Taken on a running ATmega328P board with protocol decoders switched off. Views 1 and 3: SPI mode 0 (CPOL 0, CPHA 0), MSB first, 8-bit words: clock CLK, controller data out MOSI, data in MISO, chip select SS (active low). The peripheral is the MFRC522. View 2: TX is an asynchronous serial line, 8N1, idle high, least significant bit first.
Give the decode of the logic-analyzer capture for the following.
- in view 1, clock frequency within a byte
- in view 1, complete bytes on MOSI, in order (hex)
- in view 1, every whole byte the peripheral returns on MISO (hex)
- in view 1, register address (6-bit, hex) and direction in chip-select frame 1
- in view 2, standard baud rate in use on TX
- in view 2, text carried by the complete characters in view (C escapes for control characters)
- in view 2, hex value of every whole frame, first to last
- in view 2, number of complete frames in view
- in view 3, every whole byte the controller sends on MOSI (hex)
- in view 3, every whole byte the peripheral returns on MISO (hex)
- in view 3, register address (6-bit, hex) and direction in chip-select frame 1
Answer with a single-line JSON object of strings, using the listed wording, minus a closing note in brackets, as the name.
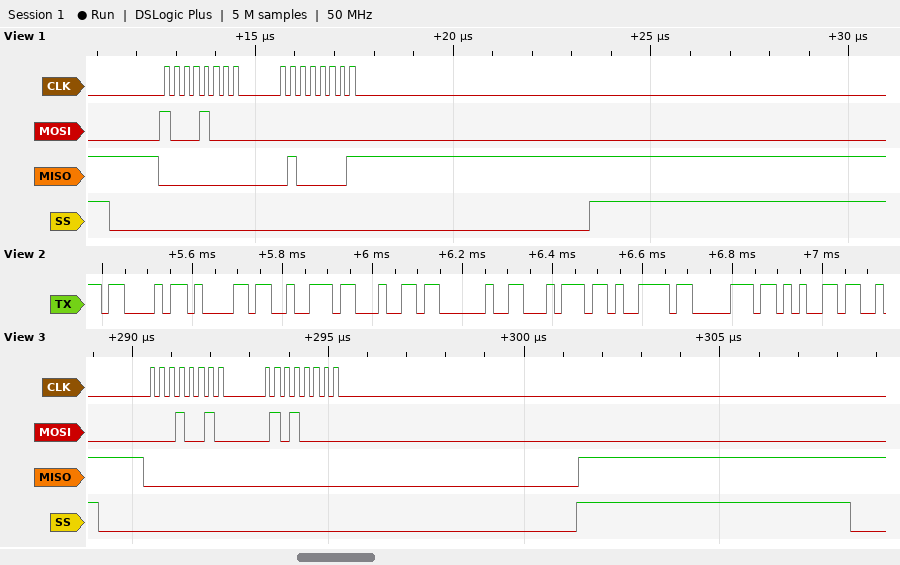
{"in view 1, clock frequency within a byte": "4 MHz", "in view 1, complete bytes on MOSI, in order": "88 00", "in view 1, every whole byte the peripheral returns on MISO": "00 41", "in view 1, register address (6-bit, hex) and direction in chip-select frame 1": "0x04 read", "in view 2, standard baud rate in use on TX": "57600 baud", "in view 2, text carried by the complete characters in view": "\"Card type\"", "in view 2, hex value of every whole frame, first to last": "43 61 72 64 20 74 79 70 65", "in view 2, number of complete frames in view": "9", "in view 3, every whole byte the controller sends on MOSI": "12 50", "in view 3, every whole byte the peripheral returns on MISO": "00 00", "in view 3, register address (6-bit, hex) and direction in chip-select frame 1": "0x09 write"}
